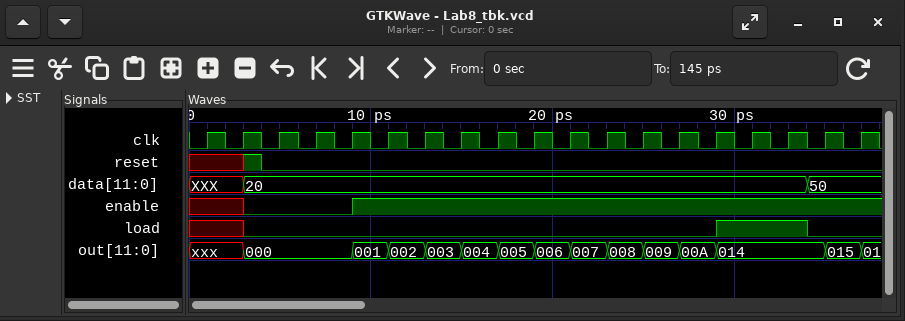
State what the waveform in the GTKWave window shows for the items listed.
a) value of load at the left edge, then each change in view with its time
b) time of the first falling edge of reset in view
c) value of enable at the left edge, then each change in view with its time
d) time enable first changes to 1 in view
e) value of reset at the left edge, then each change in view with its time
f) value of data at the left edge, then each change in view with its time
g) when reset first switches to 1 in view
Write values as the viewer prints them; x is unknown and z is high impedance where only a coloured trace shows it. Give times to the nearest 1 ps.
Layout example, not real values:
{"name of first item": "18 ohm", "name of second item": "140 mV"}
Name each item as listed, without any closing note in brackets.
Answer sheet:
{"value of load at the left edge, then each change in view with its time": "x, 0 at 3 ps, 1 at 29 ps, 0 at 34 ps", "time of the first falling edge of reset in view": "4 ps", "value of enable at the left edge, then each change in view with its time": "x, 0 at 3 ps, 1 at 9 ps", "time enable first changes to 1 in view": "9 ps", "value of reset at the left edge, then each change in view with its time": "x, 1 at 3 ps, 0 at 4 ps", "value of data at the left edge, then each change in view with its time": "XXX, 20 at 3 ps, 50 at 34 ps", "when reset first switches to 1 in view": "3 ps"}
